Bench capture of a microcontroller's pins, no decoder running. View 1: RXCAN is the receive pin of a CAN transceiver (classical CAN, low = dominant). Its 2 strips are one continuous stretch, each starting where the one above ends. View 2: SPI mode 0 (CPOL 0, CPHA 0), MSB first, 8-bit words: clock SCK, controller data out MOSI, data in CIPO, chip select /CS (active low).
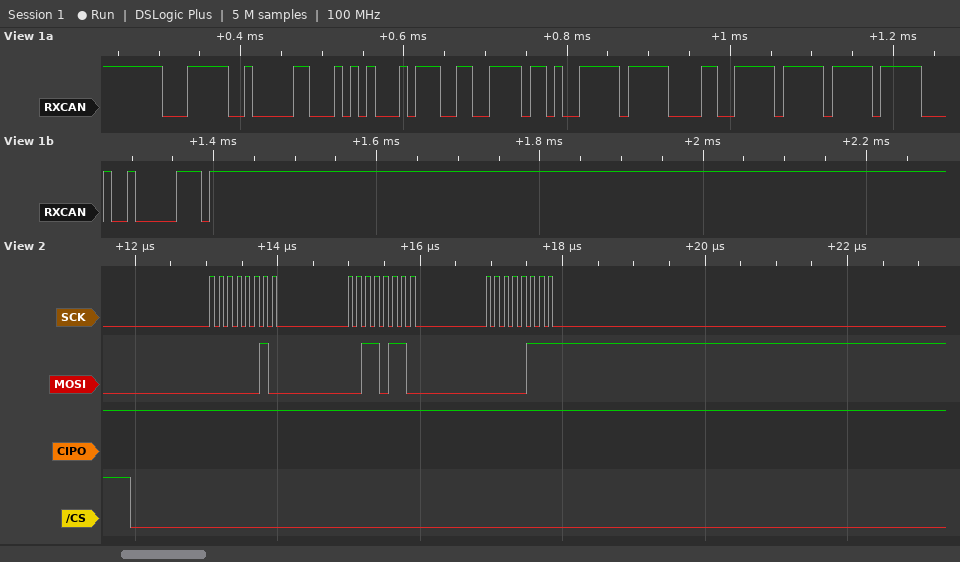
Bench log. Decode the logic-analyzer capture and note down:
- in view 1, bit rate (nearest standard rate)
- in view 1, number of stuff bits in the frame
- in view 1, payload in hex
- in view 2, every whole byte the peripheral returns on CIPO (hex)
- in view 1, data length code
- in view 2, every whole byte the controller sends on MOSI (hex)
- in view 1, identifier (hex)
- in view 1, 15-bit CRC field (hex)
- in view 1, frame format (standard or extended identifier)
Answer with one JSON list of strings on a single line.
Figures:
["100 kbit/s", "9", "A8 B9 9E D3 FF 19 FF FF", "FF FF FF", "8", "02 36 07", "0x1F4", "0x7241", "standard"]
